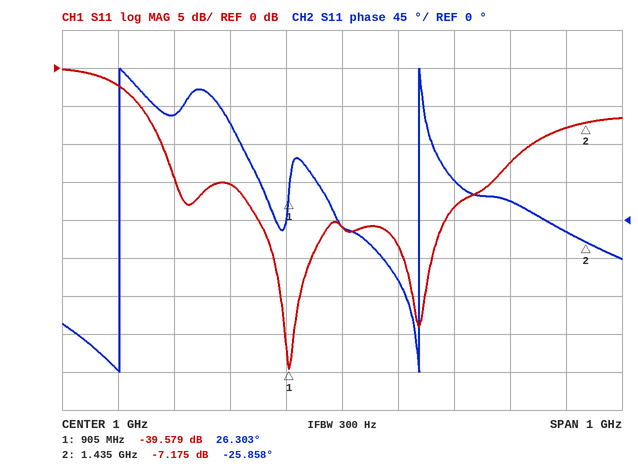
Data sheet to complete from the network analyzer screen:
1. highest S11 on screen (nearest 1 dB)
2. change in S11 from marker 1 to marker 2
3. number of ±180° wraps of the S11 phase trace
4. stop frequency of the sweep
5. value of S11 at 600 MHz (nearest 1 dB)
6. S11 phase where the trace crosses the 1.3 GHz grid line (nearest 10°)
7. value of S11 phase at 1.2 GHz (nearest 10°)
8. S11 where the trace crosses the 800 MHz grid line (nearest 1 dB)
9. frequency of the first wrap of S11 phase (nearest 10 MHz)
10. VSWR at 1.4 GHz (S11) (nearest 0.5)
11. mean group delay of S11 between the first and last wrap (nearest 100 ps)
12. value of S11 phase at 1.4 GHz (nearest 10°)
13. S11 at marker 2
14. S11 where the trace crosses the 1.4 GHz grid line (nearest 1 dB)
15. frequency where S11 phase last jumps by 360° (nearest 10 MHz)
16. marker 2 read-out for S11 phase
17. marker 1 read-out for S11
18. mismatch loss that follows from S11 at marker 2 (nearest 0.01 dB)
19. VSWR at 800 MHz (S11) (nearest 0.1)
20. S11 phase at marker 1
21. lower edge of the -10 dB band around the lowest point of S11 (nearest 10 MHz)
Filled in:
0 dB
32.404 dB
2
1.5 GHz
-2 dB
20°
50°
-15 dB
600 MHz
2.5
1.9 ns
-10°
-7.175 dB
-8 dB
1.14 GHz
-25.858°
-39.579 dB
0.92 dB
1.4
26.303°
680 MHz
